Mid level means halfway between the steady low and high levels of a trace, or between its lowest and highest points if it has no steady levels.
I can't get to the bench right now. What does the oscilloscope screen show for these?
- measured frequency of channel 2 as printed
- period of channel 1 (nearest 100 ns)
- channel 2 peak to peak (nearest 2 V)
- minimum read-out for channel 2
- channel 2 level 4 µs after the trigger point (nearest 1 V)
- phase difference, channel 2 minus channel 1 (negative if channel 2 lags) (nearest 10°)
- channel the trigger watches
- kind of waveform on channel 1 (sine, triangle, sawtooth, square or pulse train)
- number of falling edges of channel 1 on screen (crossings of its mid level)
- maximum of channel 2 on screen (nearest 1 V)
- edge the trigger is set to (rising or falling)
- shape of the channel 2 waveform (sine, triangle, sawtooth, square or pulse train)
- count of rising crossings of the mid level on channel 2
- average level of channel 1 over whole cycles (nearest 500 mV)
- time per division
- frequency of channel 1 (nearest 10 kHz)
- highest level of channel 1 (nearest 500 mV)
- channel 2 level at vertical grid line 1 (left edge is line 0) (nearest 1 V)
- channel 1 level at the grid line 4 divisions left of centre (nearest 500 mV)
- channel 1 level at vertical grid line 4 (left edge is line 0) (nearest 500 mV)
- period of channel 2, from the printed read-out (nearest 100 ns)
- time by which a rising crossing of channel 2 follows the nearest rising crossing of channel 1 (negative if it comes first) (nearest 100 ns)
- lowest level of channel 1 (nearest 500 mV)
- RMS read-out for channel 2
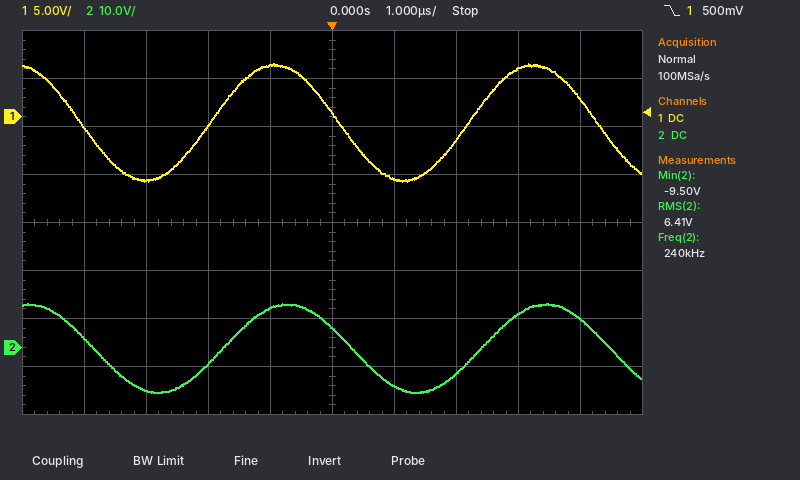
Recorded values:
240 kHz
4.2 µs
18 V
-9.50 V
6 V
-20°
channel 1
sine
3
9 V
falling
sine
2
-500 mV
1 µs
240 kHz
5.5 V
2 V
-1.0 V
5.5 V
4.2 µs
+200 ns
-6.5 V
6.41 V
